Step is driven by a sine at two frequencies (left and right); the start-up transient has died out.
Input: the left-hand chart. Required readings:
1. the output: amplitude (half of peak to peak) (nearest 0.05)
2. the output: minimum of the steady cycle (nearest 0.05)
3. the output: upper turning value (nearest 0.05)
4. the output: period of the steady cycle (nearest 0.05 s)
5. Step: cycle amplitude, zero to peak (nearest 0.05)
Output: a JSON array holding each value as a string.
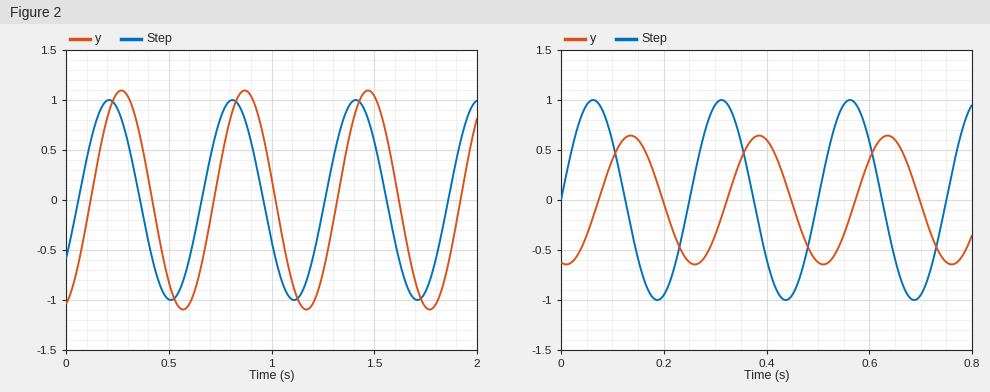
["1.10", "-1.10", "1.10", "0.60 s", "1.00"]
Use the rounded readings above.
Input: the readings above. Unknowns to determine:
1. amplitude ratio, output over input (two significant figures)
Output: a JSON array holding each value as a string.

["1.1"]
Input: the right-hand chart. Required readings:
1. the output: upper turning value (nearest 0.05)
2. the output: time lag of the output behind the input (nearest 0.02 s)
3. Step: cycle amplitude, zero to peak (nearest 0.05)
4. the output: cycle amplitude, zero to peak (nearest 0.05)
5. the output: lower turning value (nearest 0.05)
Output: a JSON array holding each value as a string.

["0.65", "0.08 s", "1.00", "0.65", "-0.65"]
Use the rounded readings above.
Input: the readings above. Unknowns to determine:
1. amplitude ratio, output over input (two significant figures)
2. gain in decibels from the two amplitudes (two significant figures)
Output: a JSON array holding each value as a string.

["0.65", "-3.7 dB"]
